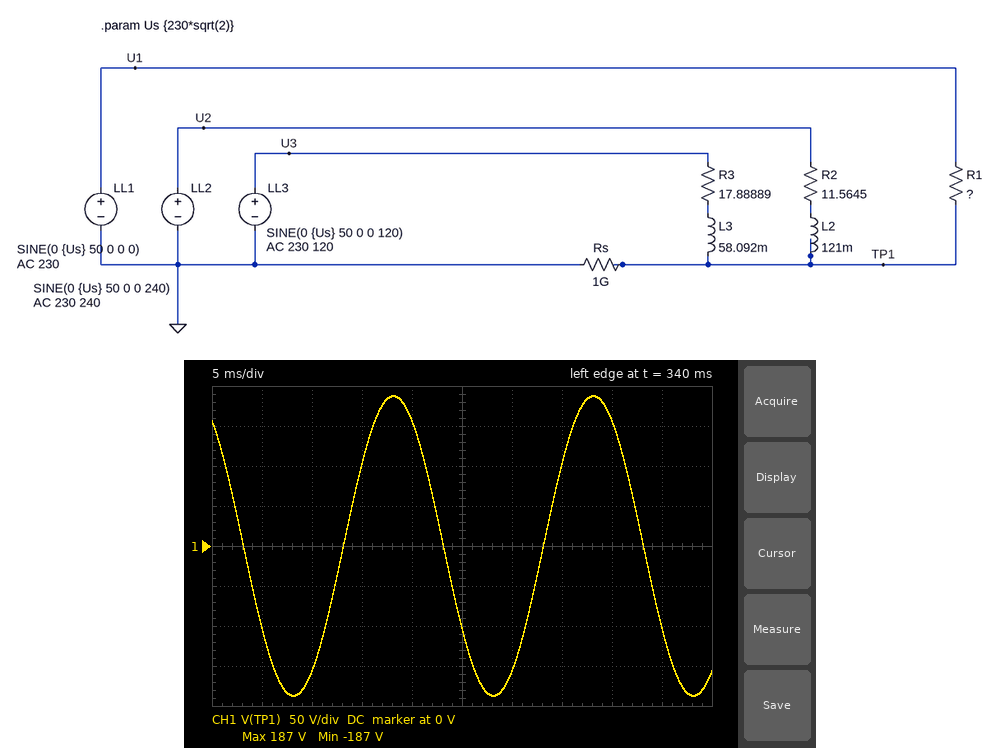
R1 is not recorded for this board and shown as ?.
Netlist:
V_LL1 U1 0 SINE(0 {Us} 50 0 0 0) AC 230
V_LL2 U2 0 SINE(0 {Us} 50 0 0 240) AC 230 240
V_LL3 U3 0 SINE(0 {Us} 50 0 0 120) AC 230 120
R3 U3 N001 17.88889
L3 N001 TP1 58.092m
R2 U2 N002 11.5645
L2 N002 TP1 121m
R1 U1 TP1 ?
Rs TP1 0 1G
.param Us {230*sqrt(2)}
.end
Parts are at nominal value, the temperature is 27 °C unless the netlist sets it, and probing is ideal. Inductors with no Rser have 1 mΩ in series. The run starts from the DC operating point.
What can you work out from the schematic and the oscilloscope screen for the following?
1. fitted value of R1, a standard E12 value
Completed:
47 Ω
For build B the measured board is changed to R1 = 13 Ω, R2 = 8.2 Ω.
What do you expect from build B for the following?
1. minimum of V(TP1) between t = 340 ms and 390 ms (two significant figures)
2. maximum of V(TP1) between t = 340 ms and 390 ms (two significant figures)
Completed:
-210 V
210 V
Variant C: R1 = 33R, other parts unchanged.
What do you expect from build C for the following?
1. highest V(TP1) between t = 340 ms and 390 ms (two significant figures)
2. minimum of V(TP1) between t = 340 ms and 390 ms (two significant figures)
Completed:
180 V
-180 V
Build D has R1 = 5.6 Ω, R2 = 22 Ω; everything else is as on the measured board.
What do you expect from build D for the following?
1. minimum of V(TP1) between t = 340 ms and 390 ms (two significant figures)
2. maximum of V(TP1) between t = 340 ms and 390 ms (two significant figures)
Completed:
-250 V
250 V
